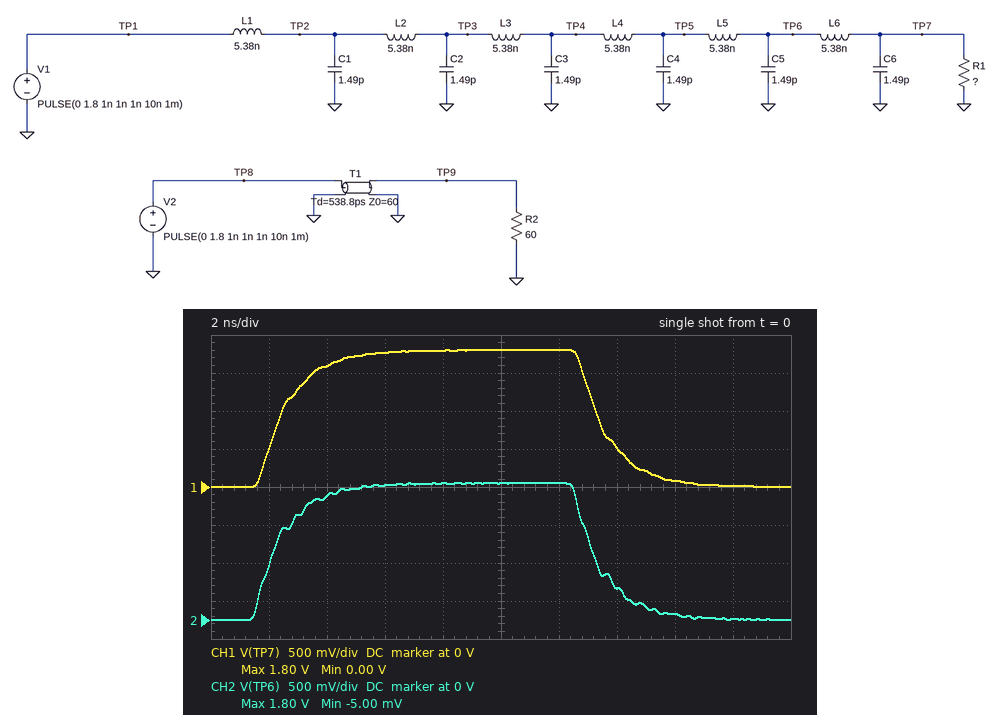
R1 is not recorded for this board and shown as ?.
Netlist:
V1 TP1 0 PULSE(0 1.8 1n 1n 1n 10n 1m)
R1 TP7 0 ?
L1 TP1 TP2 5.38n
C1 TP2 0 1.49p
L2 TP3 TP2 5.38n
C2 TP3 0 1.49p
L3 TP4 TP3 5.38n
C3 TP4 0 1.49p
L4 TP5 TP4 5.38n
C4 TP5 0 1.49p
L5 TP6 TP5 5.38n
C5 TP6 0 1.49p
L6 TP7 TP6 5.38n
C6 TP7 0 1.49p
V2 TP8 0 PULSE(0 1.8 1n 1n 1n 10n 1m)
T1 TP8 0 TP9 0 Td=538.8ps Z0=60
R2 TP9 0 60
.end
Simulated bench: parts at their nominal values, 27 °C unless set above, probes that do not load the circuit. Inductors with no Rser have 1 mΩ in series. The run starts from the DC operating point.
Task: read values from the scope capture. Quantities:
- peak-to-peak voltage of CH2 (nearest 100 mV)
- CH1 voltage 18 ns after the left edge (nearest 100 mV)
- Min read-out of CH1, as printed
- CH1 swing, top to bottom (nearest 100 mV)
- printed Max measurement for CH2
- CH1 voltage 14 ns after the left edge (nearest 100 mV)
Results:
1.8 V
0 V
0.00 V
1.8 V
1.80 V
500 mV
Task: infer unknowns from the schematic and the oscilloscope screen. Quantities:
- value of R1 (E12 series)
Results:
27 Ω
